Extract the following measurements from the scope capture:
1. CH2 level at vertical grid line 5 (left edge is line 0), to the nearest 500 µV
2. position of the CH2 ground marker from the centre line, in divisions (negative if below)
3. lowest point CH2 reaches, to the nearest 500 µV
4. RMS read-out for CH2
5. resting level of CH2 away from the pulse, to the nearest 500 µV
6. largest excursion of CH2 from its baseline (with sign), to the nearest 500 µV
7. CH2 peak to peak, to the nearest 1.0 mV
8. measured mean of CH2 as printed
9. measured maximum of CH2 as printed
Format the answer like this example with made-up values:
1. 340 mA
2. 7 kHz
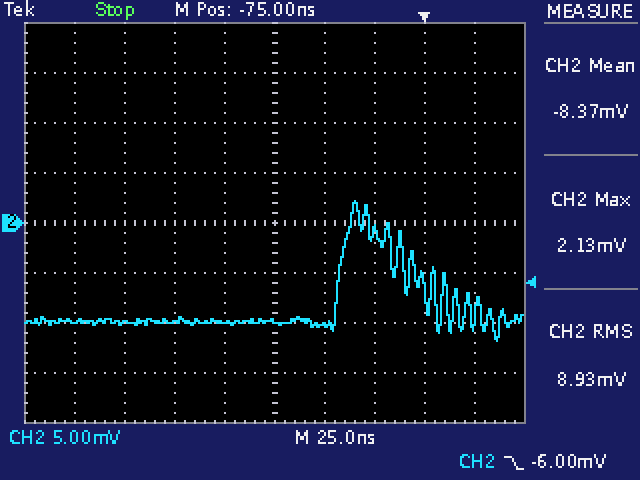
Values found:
1. -10.0 mV
2. 0.0 div
3. -12.0 mV
4. 8.93 mV
5. -10.0 mV
6. +12.0 mV
7. 14.0 mV
8. -8.37 mV
9. 2.13 mV
